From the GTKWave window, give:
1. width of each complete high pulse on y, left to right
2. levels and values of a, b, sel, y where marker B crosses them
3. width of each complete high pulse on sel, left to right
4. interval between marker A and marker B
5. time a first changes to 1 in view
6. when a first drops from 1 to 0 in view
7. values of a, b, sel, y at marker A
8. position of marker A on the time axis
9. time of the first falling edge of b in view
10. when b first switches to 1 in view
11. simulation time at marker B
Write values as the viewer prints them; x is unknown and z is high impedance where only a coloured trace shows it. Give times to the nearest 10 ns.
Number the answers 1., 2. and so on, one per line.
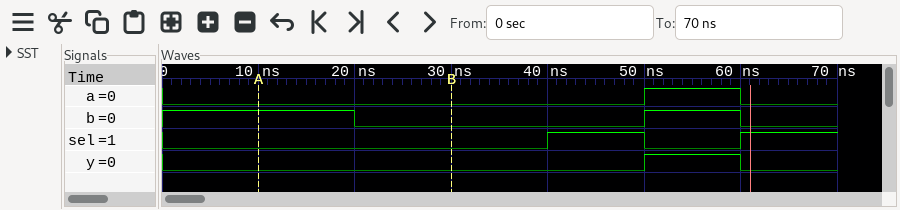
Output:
1. 10 ns
2. a=0, b=0, sel=0, y=0
3. 10 ns
4. 20 ns
5. 50 ns
6. 60 ns
7. a=0, b=1, sel=0, y=0
8. 10 ns
9. 20 ns
10. 50 ns
11. 30 ns
